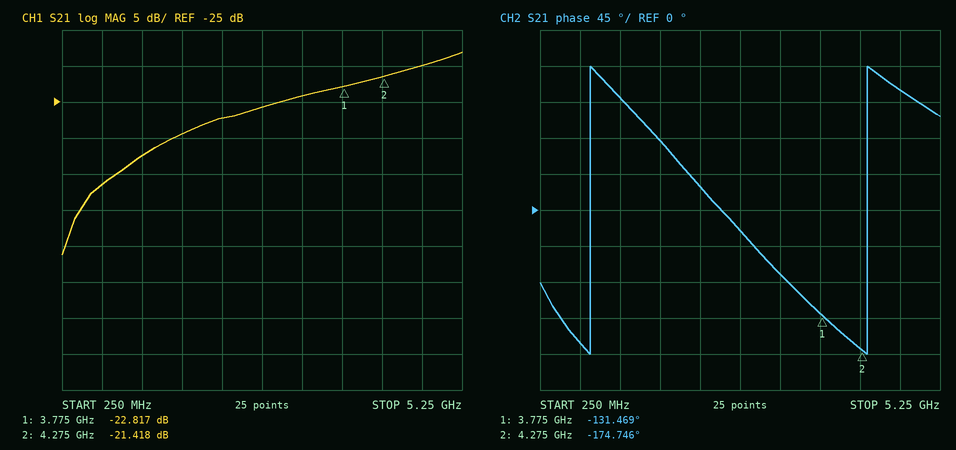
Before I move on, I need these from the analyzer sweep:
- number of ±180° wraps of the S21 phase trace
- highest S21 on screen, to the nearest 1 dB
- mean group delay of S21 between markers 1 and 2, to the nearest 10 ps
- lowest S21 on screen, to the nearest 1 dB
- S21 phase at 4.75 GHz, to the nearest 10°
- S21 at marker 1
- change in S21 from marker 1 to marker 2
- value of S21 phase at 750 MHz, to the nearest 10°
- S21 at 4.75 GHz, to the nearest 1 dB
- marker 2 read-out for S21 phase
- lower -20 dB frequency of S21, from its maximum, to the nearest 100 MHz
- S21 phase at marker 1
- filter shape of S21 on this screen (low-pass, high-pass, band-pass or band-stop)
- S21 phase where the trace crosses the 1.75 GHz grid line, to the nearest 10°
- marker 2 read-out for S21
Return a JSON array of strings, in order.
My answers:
["2", "-18 dB", "240 ps", "-46 dB", "150°", "-22.817 dB", "1.399 dB", "-170°", "-20 dB", "-174.746°", "600 MHz", "-131.469°", "high-pass", "90°", "-21.418 dB"]
